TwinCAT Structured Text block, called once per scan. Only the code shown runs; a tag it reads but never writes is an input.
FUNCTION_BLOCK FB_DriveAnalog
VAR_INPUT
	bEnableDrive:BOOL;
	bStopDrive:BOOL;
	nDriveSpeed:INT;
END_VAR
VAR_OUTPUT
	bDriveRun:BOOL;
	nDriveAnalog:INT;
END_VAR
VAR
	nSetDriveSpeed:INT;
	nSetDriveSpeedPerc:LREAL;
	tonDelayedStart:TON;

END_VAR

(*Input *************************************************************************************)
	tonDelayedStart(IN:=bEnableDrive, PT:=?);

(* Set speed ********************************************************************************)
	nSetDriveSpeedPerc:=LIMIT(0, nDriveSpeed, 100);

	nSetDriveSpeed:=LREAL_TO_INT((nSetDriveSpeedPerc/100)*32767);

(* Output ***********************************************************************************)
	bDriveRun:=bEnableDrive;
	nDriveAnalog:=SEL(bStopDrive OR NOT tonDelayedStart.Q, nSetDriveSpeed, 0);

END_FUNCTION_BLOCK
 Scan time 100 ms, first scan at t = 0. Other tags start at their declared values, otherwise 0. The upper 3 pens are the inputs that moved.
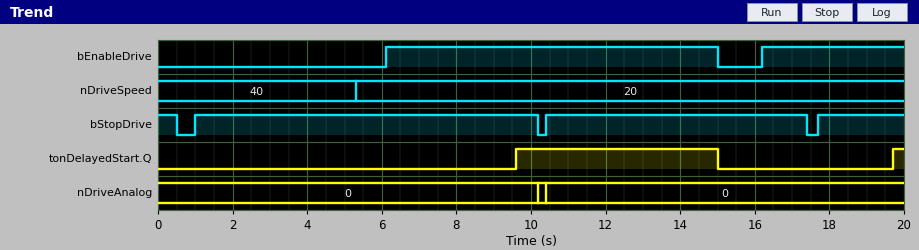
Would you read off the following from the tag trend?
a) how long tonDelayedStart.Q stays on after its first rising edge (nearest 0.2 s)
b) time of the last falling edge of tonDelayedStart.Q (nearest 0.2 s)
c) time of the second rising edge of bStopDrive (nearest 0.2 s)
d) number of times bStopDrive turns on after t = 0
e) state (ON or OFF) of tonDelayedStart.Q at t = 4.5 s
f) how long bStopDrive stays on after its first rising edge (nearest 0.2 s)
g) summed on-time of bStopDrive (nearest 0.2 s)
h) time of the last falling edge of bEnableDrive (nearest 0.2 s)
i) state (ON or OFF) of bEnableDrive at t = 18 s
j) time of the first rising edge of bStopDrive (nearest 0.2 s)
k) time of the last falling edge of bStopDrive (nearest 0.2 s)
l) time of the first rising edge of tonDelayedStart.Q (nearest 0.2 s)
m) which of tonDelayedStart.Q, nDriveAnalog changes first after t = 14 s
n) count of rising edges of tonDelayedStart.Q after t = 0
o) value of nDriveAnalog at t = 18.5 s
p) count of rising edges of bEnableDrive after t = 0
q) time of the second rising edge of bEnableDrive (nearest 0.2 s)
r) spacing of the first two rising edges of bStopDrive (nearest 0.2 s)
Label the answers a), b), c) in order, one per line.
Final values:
a) 5.4 s
b) 15.0 s
c) 10.4 s
d) 3
e) OFF
f) 9.2 s
g) 19.0 s
h) 15.0 s
i) ON
j) 1.0 s
k) 17.4 s
l) 9.6 s
m) tonDelayedStart.Q
n) 2
o) 0
p) 2
q) 16.2 s
r) 9.4 s
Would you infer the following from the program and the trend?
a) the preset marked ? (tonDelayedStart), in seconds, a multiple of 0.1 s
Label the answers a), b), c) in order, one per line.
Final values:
a) 3.5 s
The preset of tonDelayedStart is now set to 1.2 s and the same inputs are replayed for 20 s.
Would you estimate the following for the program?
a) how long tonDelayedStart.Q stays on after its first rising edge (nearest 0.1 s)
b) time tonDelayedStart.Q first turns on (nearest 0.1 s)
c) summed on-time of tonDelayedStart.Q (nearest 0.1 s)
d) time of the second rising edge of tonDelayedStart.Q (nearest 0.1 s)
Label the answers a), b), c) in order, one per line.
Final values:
a) 7.7 s
b) 7.3 s
c) 10.3 s
d) 17.4 s
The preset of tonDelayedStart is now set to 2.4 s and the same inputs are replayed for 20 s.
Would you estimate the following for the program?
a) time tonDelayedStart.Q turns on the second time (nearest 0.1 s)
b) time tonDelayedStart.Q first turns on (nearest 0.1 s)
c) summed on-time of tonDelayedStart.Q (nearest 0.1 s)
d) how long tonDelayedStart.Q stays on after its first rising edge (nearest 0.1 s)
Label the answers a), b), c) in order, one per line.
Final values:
a) 18.6 s
b) 8.5 s
c) 7.9 s
d) 6.5 s
